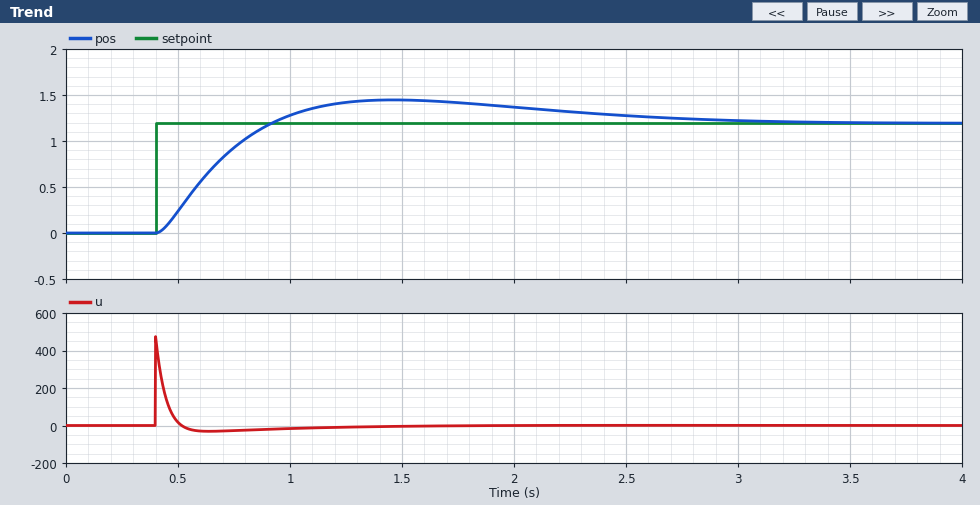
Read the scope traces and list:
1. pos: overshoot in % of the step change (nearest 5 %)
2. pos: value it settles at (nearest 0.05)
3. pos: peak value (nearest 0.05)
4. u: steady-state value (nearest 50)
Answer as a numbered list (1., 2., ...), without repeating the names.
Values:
1. 20 %
2. 1.20
3. 1.45
4. 0
